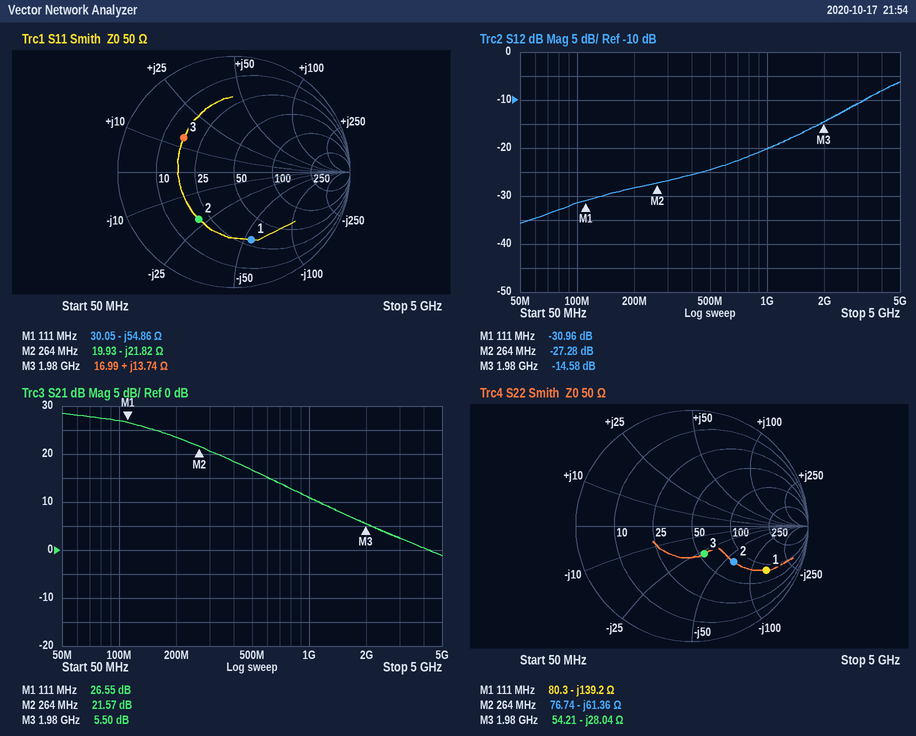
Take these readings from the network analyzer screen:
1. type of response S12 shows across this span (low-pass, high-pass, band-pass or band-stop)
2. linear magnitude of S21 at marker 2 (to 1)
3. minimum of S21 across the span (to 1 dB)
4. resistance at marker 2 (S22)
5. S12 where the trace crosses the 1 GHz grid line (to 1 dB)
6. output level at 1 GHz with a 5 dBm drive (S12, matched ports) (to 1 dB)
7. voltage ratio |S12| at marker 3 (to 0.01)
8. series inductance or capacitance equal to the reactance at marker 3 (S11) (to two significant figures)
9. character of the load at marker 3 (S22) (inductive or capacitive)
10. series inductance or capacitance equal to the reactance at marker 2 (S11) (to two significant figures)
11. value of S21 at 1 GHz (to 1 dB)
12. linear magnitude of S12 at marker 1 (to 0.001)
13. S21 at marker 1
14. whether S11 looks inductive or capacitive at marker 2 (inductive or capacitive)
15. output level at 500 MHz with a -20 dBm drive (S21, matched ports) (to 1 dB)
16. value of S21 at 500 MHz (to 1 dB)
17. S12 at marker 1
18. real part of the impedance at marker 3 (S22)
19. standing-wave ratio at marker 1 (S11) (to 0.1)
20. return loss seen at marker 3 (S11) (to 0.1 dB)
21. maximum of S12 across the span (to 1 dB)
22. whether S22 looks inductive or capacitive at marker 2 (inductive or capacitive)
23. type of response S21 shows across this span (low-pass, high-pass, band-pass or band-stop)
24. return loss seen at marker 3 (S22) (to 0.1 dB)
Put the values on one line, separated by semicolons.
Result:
high-pass; 12; -1 dB; 76.74 Ω; -20 dB; -15 dBm; 0.19; 1.1 nH; capacitive; 28 pF; 11 dB; 0.028; 26.55 dB; capacitive; -3 dBm; 17 dB; -30.96 dB; 54.21 Ω; 4.0; 5.6 dB; -6 dB; capacitive; low-pass; 11.6 dB
